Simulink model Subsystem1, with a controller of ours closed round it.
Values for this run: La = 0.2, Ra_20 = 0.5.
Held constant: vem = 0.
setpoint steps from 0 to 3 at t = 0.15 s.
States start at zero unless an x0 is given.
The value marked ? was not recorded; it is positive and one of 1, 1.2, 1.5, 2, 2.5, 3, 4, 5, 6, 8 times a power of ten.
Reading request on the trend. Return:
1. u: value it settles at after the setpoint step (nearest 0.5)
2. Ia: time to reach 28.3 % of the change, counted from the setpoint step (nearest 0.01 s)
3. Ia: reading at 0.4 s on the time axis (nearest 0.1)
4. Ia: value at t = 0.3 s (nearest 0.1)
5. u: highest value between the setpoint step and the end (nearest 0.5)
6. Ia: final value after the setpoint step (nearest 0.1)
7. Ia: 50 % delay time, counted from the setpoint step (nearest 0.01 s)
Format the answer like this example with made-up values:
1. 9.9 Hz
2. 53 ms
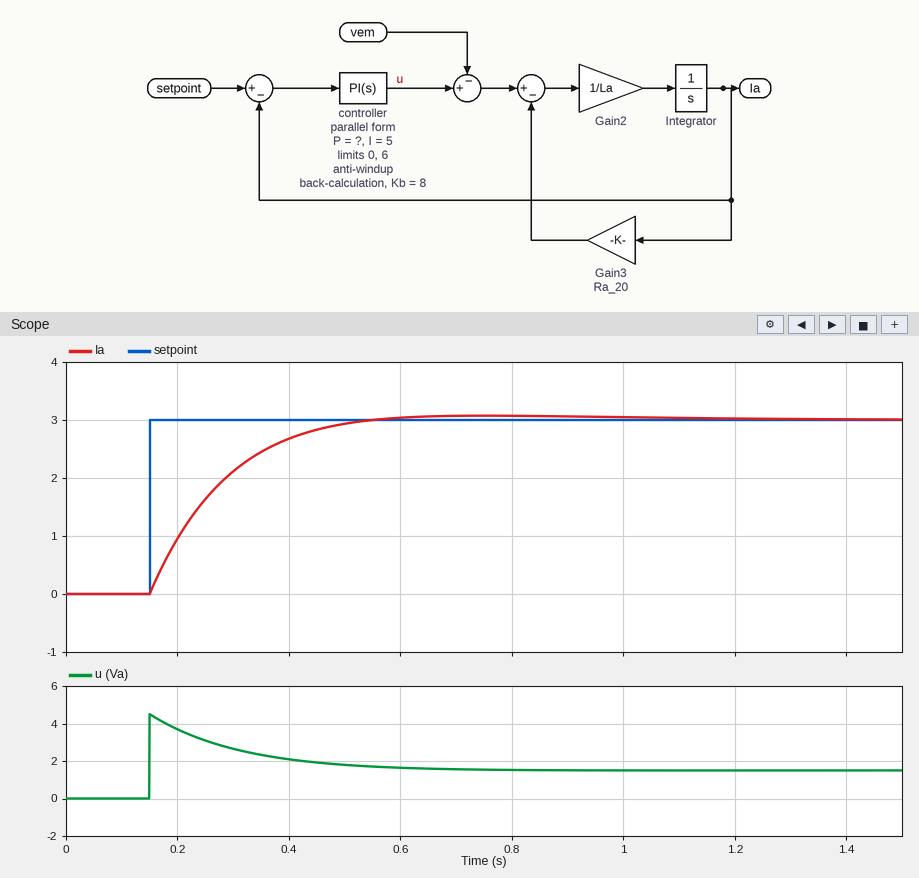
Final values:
1. 1.5
2. 0.04 s
3. 2.7
4. 2.1
5. 4.5
6. 3.0
7. 0.09 s
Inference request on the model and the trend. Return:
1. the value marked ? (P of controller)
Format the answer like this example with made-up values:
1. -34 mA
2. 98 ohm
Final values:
1. 1.5
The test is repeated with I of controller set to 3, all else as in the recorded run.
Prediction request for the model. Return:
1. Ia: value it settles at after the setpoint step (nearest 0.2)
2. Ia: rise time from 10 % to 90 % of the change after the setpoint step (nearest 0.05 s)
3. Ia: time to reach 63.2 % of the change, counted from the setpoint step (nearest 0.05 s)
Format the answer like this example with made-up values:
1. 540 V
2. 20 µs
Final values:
1. 3.0
2. 0.35 s
3. 0.15 s
